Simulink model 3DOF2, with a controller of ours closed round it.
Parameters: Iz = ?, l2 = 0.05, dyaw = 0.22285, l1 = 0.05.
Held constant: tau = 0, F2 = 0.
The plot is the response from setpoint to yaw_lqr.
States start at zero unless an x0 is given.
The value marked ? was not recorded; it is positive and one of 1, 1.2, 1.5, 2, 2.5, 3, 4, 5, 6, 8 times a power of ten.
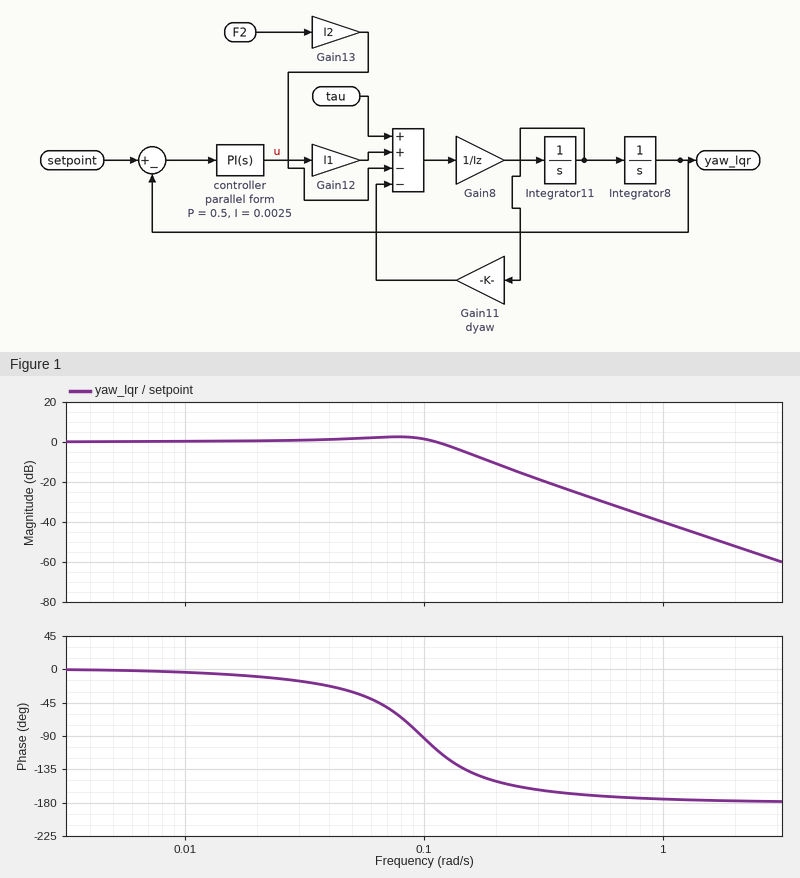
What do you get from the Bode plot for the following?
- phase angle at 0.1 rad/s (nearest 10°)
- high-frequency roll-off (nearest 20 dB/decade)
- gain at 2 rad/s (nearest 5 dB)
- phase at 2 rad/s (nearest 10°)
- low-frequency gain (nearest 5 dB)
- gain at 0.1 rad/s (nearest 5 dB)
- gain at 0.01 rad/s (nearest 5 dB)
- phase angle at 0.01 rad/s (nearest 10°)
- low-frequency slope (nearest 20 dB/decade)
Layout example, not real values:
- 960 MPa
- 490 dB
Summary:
- -90°
- -40 dB/decade
- -50 dB
- -180°
- 0 dB
- 0 dB
- 0 dB
- 0°
- 0 dB/decade
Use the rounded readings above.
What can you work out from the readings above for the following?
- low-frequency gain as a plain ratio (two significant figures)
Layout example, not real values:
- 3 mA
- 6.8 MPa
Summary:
- 1.0
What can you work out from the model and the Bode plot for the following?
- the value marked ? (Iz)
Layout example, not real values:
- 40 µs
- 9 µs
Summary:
- 2.5
